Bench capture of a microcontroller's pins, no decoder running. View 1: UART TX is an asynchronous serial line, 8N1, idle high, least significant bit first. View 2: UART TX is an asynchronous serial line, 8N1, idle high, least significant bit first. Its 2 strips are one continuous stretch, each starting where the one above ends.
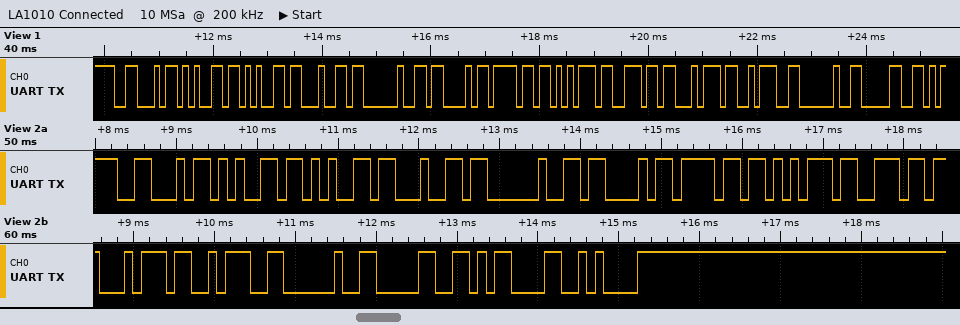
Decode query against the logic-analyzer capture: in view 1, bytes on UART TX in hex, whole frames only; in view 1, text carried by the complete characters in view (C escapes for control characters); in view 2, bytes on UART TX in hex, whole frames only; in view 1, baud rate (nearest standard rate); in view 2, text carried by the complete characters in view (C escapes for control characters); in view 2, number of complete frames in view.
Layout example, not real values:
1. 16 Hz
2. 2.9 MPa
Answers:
1. 0x46 0x65 0x65 0x64 0x20 0x43 0x6F 0x75 0x6E 0x74 0x3A 0x20 0x30
2. "Feed Count: 0"
3. 46 65 65 64 20 43 6F 75 6E 74 3A 20 30 0D 0A
4. 9600 baud
5. "Feed Count: 0\r\n"
6. 15
